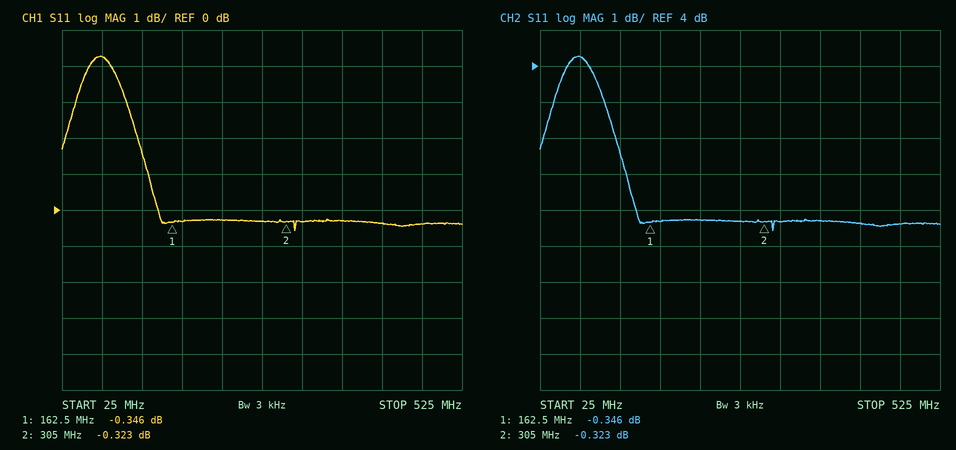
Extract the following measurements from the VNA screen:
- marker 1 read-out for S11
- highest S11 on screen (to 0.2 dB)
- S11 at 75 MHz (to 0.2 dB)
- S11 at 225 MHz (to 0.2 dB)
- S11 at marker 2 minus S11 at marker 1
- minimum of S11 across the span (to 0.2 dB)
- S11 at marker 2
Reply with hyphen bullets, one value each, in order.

- -0.346 dB
- 4.2 dB
- 4.2 dB
- -0.2 dB
- 0.023 dB
- -0.6 dB
- -0.323 dB
